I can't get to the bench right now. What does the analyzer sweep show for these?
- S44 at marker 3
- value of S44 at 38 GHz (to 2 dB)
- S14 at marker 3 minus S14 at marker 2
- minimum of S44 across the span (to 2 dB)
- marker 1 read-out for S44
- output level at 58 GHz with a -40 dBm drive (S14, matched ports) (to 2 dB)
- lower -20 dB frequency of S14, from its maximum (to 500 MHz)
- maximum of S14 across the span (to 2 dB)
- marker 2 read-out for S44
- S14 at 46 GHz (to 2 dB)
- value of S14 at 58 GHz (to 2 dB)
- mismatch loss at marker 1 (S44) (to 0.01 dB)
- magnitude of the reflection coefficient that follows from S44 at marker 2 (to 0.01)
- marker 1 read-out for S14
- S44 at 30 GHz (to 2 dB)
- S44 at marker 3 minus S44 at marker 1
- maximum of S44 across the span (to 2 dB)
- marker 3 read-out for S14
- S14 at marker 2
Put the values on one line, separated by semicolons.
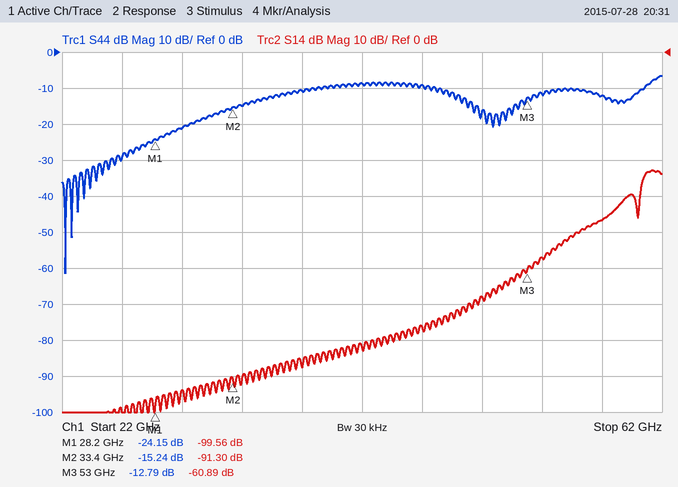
-12.79 dB; -10 dB; 30.41 dB; -62 dB; -24.15 dB; -86 dBm; 55.5 GHz; -32 dB; -15.24 dB; -76 dB; -46 dB; 0.02 dB; 0.17; -99.56 dB; -22 dB; 11.36 dB; -6 dB; -60.89 dB; -91.30 dB
